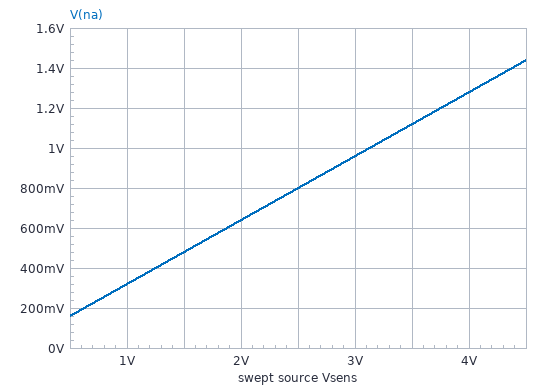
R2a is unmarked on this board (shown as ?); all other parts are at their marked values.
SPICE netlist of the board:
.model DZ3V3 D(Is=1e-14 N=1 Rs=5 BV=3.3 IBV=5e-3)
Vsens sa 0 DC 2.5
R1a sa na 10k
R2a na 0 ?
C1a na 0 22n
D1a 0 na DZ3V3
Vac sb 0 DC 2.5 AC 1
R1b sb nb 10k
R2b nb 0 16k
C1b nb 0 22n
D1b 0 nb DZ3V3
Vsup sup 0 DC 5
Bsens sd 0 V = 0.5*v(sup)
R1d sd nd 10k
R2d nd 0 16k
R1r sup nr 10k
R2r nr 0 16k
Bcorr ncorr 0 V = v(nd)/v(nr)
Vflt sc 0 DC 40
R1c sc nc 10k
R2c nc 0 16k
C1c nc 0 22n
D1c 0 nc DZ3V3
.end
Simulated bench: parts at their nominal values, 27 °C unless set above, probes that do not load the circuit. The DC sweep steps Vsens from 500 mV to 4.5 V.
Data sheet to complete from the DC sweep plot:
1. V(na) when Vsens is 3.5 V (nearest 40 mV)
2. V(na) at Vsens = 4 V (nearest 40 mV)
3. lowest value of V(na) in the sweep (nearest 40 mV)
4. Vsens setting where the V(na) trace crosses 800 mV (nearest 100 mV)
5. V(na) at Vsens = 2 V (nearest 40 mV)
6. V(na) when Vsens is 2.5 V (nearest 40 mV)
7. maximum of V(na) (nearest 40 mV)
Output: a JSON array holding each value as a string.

["1.12 V", "1.28 V", "160 mV", "2.5 V", "640 mV", "800 mV", "1.44 V"]
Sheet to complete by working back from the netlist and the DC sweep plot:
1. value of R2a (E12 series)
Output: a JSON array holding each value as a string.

["4.7 kΩ"]
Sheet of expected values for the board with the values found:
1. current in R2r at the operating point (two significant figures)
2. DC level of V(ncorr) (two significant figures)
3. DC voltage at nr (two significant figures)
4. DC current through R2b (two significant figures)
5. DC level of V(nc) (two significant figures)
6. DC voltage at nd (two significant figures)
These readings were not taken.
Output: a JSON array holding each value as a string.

["190 µA", "500 mV", "3.1 V", "96 µA", "3.3 V", "1.5 V"]
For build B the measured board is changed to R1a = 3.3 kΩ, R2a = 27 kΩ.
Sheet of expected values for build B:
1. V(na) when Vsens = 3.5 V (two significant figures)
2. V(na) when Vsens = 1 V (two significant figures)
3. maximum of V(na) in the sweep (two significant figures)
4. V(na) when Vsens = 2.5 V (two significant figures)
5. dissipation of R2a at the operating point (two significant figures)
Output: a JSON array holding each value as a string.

["3.1 V", "890 mV", "3.2 V", "2.2 V", "180 µW"]
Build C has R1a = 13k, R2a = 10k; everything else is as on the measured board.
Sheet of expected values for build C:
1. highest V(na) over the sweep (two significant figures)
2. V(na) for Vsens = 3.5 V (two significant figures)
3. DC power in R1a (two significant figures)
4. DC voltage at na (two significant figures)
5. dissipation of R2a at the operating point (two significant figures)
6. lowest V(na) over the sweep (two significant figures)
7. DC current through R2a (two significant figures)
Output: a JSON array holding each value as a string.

["2.0 V", "1.5 V", "150 µW", "1.1 V", "120 µW", "220 mV", "110 µA"]
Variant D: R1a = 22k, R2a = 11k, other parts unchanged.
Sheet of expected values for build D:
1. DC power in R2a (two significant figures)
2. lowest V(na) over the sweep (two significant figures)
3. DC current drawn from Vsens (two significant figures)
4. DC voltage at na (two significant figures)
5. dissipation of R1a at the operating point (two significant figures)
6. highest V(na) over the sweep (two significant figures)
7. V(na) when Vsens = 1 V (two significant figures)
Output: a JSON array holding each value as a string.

["63 µW", "170 mV", "76 µA", "830 mV", "130 µW", "1.5 V", "330 mV"]
